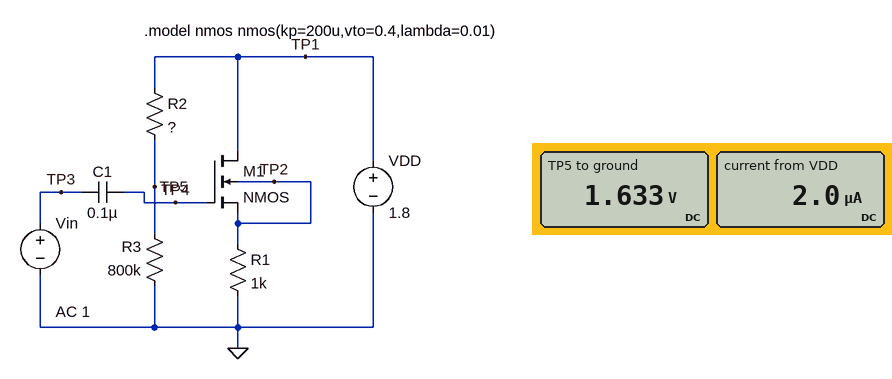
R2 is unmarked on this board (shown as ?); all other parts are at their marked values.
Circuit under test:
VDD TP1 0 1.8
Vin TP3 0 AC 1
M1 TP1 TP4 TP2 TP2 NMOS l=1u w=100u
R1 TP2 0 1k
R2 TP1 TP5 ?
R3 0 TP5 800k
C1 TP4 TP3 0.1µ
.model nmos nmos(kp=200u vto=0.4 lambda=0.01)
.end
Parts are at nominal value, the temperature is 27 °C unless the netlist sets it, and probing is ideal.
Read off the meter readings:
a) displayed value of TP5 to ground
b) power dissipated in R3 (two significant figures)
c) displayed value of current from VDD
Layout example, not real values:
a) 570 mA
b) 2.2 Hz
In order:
a) 1.633 V
b) 3.3 µW
c) 2.0 µA
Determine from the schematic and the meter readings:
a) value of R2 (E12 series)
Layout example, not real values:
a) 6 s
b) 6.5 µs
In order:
a) 82 kΩ
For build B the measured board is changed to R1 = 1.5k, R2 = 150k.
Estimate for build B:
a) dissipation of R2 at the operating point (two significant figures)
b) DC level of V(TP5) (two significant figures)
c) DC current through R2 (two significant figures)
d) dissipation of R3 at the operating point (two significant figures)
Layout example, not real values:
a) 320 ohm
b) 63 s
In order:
a) 540 nW
b) 1.5 V
c) 1.9 µA
d) 2.9 µW
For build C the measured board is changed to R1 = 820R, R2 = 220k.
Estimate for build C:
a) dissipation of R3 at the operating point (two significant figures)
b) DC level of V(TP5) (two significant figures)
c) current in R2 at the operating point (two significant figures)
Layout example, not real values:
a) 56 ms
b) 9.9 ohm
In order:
a) 2.5 µW
b) 1.4 V
c) 1.8 µA
